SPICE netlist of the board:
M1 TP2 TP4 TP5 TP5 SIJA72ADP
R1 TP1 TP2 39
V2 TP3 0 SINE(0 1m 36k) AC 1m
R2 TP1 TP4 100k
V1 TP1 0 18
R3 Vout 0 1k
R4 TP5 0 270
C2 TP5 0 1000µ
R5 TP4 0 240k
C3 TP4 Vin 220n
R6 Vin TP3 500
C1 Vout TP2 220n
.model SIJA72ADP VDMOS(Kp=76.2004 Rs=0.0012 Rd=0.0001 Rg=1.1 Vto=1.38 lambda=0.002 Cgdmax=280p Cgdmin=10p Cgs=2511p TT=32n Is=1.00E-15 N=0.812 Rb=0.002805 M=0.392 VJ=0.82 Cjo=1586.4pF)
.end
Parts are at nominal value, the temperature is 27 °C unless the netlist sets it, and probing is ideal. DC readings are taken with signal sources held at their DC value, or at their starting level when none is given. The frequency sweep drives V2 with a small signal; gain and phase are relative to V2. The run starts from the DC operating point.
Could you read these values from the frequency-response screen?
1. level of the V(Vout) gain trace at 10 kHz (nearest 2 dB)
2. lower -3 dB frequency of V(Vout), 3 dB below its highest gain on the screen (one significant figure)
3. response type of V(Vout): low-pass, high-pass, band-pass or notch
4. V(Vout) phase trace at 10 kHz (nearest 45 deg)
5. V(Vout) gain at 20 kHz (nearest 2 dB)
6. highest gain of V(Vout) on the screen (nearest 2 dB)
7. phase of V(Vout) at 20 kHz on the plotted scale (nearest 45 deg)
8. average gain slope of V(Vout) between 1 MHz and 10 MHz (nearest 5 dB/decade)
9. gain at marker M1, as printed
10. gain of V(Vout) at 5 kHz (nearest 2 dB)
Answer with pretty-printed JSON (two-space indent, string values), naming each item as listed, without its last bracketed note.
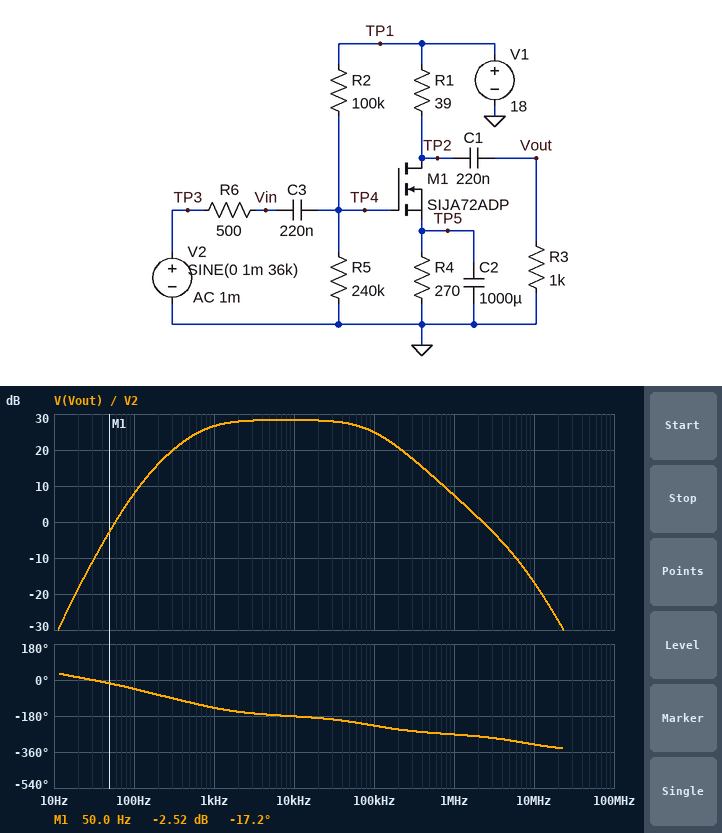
{
  "level of the V(Vout) gain trace at 10 kHz": "28 dB",
  "lower -3 dB frequency of V(Vout), 3 dB below its highest gain on the screen": "700 Hz",
  "response type of V(Vout): low-pass, high-pass, band-pass or notch": "band-pass",
  "V(Vout) phase trace at 10 kHz": "-180 deg",
  "V(Vout) gain at 20 kHz": "28 dB",
  "highest gain of V(Vout) on the screen": "28 dB",
  "phase of V(Vout) at 20 kHz on the plotted scale": "-180 deg",
  "average gain slope of V(Vout) between 1 MHz and 10 MHz": "-25 dB/decade",
  "gain at marker M1, as printed": "-2.52 dB",
  "gain of V(Vout) at 5 kHz": "28 dB"
}
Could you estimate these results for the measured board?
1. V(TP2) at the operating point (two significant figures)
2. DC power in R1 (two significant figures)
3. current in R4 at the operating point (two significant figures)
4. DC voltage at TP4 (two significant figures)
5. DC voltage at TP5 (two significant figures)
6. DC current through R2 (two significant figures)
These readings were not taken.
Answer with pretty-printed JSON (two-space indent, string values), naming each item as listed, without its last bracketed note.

{
  "V(TP2) at the operating point": "16 V",
  "DC power in R1": "70 mW",
  "current in R4 at the operating point": "42 mA",
  "DC voltage at TP4": "13 V",
  "DC voltage at TP5": "11 V",
  "DC current through R2": "53 µA"
}
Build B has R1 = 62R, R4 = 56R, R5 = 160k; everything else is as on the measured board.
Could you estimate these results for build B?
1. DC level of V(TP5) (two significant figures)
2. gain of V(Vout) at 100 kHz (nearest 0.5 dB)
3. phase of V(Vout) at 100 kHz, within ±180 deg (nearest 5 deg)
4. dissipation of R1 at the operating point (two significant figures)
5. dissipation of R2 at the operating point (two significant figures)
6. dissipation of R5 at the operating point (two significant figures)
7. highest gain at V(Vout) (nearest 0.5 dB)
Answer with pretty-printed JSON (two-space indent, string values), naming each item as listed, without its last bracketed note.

{
  "DC level of V(TP5)": "8.5 V",
  "gain of V(Vout) at 100 kHz": "-59.0 dB",
  "phase of V(Vout) at 100 kHz, within ±180 deg": "140 deg",
  "dissipation of R1 at the operating point": "1.4 W",
  "dissipation of R2 at the operating point": "480 µW",
  "dissipation of R5 at the operating point": "770 µW",
  "highest gain at V(Vout)": "-56.5 dB"
}
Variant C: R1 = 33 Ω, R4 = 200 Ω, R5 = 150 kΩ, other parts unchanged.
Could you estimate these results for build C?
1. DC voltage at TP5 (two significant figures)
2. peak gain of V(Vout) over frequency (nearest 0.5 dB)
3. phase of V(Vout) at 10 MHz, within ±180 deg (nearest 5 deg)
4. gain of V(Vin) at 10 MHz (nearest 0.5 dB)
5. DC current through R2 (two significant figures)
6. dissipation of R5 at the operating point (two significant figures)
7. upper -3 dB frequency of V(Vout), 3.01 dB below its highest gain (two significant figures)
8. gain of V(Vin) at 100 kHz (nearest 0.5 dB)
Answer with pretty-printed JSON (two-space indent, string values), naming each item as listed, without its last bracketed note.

{
  "DC voltage at TP5": "9.5 V",
  "peak gain of V(Vout) over frequency": "28.0 dB",
  "phase of V(Vout) at 10 MHz, within ±180 deg": "45 deg",
  "gain of V(Vin) at 10 MHz": "-38.5 dB",
  "DC current through R2": "72 µA",
  "dissipation of R5 at the operating point": "780 µW",
  "upper -3 dB frequency of V(Vout), 3.01 dB below its highest gain": "100 kHz",
  "gain of V(Vin) at 100 kHz": "-3.0 dB"
}
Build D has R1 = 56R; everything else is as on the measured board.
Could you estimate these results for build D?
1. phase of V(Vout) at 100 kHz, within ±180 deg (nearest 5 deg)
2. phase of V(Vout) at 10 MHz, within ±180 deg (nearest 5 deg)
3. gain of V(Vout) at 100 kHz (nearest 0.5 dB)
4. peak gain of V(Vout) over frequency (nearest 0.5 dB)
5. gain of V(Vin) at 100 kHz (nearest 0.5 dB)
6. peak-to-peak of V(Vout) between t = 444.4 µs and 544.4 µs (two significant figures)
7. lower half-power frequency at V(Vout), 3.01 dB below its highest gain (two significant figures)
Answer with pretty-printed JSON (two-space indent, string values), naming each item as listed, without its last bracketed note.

{
  "phase of V(Vout) at 100 kHz, within ±180 deg": "125 deg",
  "phase of V(Vout) at 10 MHz, within ±180 deg": "30 deg",
  "gain of V(Vout) at 100 kHz": "27.0 dB",
  "peak gain of V(Vout) over frequency": "31.5 dB",
  "gain of V(Vin) at 100 kHz": "-4.5 dB",
  "peak-to-peak of V(Vout) between t = 444.4 µs and 544.4 µs": "67 mV",
  "lower half-power frequency at V(Vout), 3.01 dB below its highest gain": "690 Hz"
}
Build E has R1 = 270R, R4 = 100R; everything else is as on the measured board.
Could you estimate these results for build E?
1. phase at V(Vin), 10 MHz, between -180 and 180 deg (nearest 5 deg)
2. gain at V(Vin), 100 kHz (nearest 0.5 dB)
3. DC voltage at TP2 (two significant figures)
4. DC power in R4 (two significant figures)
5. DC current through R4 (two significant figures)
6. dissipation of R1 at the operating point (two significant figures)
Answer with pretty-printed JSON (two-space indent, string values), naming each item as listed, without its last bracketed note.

{
  "phase at V(Vin), 10 MHz, between -180 and 180 deg": "-80 deg",
  "gain at V(Vin), 100 kHz": "-2.5 dB",
  "DC voltage at TP2": "4.9 V",
  "DC power in R4": "240 mW",
  "DC current through R4": "49 mA",
  "dissipation of R1 at the operating point": "640 mW"
}
